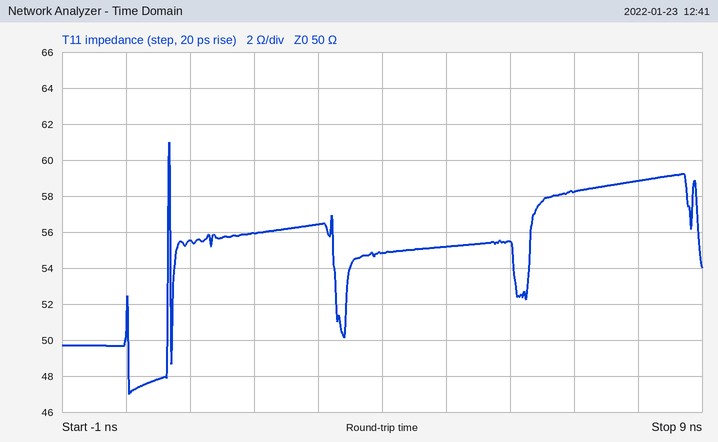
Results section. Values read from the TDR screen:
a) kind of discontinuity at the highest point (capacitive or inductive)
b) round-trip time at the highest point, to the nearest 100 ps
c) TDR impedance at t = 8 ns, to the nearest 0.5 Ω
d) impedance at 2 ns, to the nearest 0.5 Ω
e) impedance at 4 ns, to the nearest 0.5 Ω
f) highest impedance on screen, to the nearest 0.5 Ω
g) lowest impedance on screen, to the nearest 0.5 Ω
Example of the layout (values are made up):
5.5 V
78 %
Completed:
inductive
700 ps
59.0 Ω
56.0 Ω
55.0 Ω
61.0 Ω
47.0 Ω
